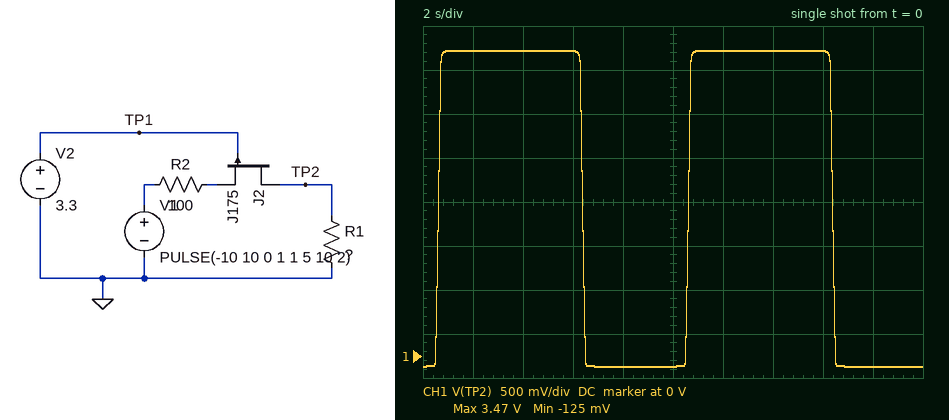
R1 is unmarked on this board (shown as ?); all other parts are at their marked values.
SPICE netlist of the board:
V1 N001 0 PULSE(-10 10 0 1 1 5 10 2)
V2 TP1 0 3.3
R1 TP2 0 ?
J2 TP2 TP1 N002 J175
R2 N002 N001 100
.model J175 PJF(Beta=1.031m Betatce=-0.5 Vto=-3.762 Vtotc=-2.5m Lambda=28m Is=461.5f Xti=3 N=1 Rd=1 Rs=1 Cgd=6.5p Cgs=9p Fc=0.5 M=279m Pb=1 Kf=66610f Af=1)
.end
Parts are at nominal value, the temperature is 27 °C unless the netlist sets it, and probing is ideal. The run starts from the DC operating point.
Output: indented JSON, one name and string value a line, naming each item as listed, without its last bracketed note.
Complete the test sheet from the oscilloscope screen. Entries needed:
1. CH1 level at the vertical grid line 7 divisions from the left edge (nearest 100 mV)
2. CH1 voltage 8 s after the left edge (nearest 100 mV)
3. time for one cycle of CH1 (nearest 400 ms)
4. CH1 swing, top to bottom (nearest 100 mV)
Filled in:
{
  "CH1 level at the vertical grid line 7 divisions from the left edge": "3.5 V",
  "CH1 voltage 8 s after the left edge": "-100 mV",
  "time for one cycle of CH1": "10.0 s",
  "CH1 swing, top to bottom": "3.6 V"
}
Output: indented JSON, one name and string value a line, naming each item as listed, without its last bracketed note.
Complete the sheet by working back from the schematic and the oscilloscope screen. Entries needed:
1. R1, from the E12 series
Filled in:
{
  "R1, from the E12 series": "820 Ω"
}
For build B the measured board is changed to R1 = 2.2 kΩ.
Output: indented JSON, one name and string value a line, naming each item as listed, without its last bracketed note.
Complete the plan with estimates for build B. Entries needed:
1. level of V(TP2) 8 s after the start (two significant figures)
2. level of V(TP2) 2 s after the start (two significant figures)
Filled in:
{
  "level of V(TP2) 8 s after the start": "-200 mV",
  "level of V(TP2) 2 s after the start": "3.8 V"
}
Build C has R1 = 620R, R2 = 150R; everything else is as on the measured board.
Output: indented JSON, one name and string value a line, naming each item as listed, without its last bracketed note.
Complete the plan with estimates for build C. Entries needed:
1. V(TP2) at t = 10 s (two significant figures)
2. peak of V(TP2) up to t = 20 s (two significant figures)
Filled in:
{
  "V(TP2) at t = 10 s": "-100 mV",
  "peak of V(TP2) up to t = 20 s": "3.3 V"
}
